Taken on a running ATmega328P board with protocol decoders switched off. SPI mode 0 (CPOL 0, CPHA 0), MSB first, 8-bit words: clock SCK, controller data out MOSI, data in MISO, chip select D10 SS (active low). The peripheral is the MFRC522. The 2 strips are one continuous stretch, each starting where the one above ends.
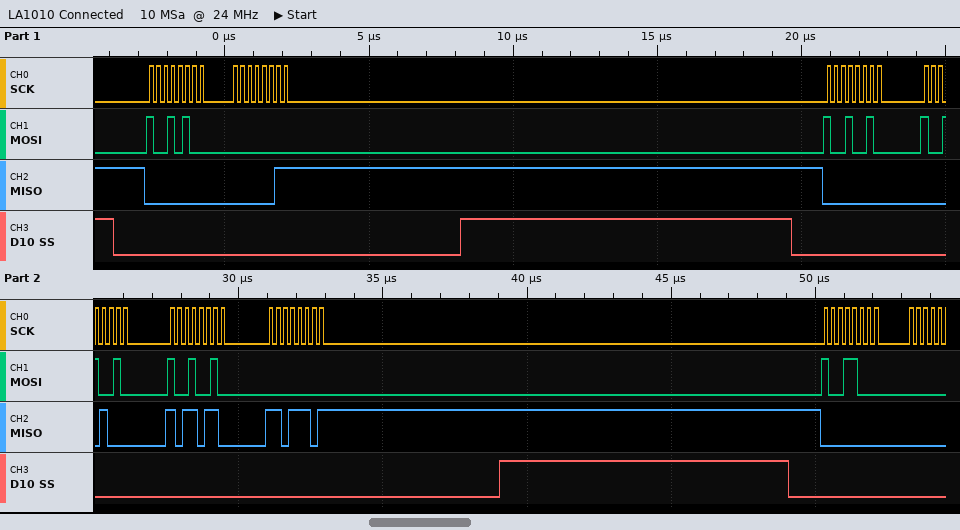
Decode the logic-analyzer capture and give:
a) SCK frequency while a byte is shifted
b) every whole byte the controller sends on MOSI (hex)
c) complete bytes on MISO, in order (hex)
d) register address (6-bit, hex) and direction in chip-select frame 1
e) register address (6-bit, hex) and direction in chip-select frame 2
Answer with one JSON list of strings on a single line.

["4 MHz", "94 00 92 92 92 00 98", "00 03 00 08 B6 DD 00", "0x0A read", "0x09 read"]
